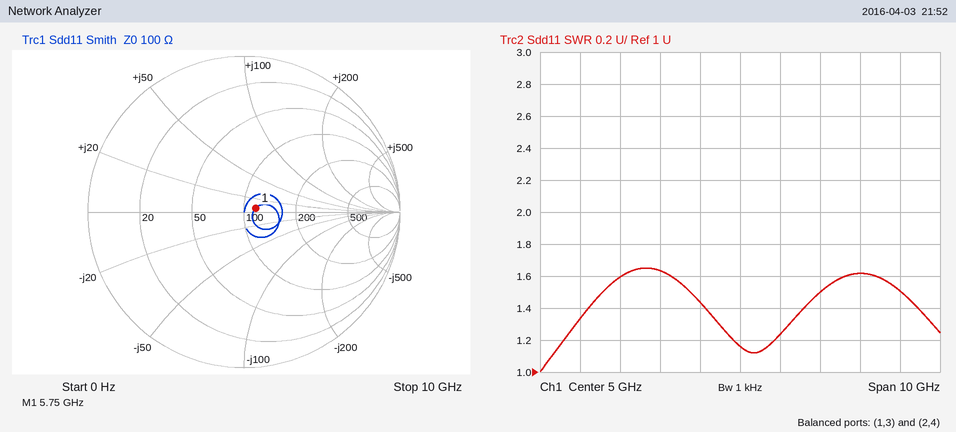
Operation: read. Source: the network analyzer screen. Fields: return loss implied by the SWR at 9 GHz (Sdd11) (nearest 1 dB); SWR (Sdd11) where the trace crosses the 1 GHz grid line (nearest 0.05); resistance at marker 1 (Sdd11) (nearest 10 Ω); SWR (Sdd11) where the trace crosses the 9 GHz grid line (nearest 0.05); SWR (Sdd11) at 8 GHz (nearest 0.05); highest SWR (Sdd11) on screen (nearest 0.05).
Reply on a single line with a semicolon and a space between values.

14 dB; 1.35; 120 Ω; 1.50; 1.60; 1.65
